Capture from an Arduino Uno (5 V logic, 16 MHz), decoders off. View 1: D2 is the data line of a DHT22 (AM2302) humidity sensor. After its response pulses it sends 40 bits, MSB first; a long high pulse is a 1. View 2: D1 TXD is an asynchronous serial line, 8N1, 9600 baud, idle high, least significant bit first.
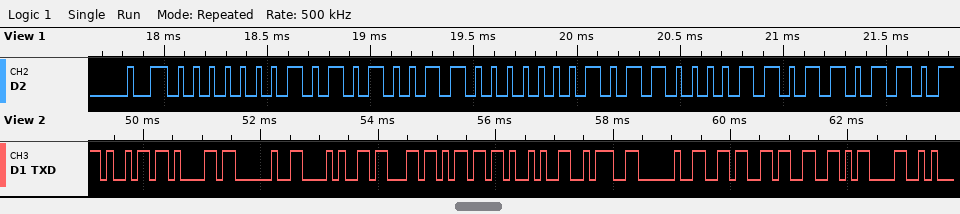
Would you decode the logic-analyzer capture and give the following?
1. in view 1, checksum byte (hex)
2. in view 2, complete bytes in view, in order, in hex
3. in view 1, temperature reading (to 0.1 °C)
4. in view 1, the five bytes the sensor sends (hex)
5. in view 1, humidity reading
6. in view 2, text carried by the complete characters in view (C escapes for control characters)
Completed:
0xB6
69 61 20 28 63 6D 29 3A 20 36 33 0D
35.3 °C
01 53 01 61 B6
33.9 %
"ia (cm): 63\r"
